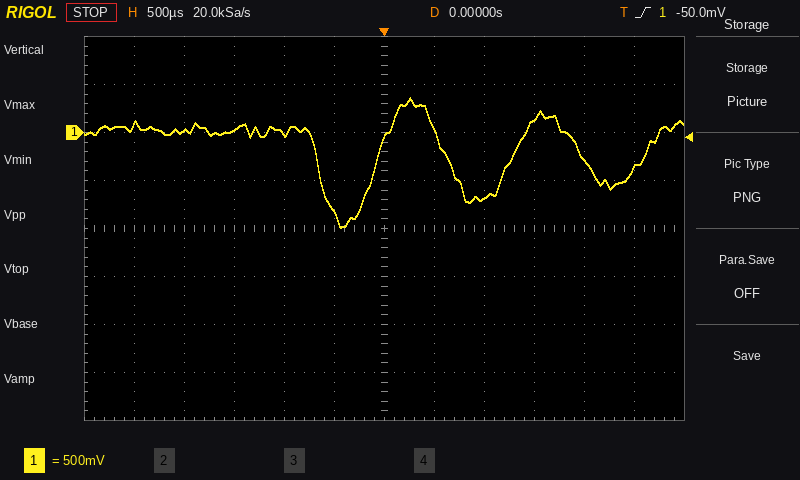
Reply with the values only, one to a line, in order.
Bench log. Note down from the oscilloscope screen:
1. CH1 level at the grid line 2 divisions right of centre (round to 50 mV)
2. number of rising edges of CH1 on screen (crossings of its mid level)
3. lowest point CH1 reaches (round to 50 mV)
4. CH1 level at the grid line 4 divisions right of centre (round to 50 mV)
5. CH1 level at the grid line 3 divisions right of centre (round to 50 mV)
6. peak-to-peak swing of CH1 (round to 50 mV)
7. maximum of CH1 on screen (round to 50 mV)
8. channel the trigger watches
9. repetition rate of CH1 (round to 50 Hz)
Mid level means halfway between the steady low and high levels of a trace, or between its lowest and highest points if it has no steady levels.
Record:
-700 mV
3
-1.00 V
-300 mV
150 mV
1.35 V
350 mV
CH1
750 Hz
